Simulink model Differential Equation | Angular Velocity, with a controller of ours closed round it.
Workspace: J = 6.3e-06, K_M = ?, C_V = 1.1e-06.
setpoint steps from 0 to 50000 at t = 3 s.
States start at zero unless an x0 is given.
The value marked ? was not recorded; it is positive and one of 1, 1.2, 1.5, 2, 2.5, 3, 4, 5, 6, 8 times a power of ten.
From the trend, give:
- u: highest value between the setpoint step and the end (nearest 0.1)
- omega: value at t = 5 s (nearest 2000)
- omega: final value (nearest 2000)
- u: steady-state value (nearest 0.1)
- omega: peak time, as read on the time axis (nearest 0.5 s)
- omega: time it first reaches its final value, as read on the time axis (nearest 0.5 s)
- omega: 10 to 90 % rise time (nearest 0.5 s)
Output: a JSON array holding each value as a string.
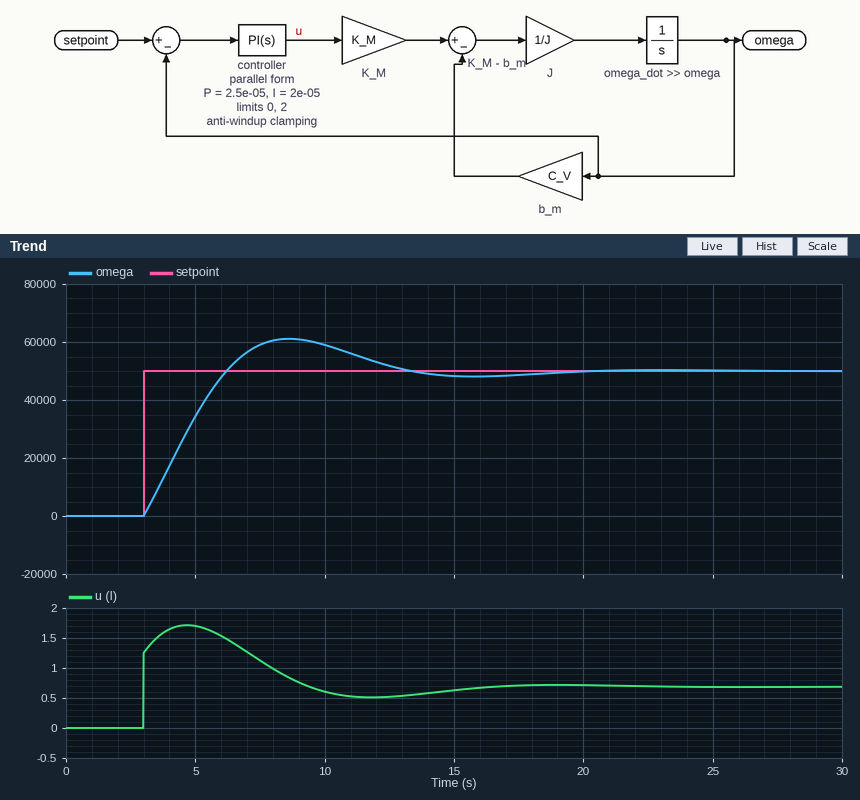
["1.7", "34000", "50000", "0.7", "8.5 s", "6.0 s", "2.5 s"]
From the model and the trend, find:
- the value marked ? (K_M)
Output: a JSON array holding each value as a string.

["0.08"]
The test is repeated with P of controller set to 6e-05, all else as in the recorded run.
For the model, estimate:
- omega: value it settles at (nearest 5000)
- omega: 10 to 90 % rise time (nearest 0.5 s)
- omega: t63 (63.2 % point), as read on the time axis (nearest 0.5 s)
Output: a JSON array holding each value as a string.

["50000", "3.0 s", "4.5 s"]
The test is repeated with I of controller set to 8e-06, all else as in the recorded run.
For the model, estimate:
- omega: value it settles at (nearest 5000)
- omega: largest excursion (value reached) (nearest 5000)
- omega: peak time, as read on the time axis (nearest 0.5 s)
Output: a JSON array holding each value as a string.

["50000", "55000", "12.5 s"]
